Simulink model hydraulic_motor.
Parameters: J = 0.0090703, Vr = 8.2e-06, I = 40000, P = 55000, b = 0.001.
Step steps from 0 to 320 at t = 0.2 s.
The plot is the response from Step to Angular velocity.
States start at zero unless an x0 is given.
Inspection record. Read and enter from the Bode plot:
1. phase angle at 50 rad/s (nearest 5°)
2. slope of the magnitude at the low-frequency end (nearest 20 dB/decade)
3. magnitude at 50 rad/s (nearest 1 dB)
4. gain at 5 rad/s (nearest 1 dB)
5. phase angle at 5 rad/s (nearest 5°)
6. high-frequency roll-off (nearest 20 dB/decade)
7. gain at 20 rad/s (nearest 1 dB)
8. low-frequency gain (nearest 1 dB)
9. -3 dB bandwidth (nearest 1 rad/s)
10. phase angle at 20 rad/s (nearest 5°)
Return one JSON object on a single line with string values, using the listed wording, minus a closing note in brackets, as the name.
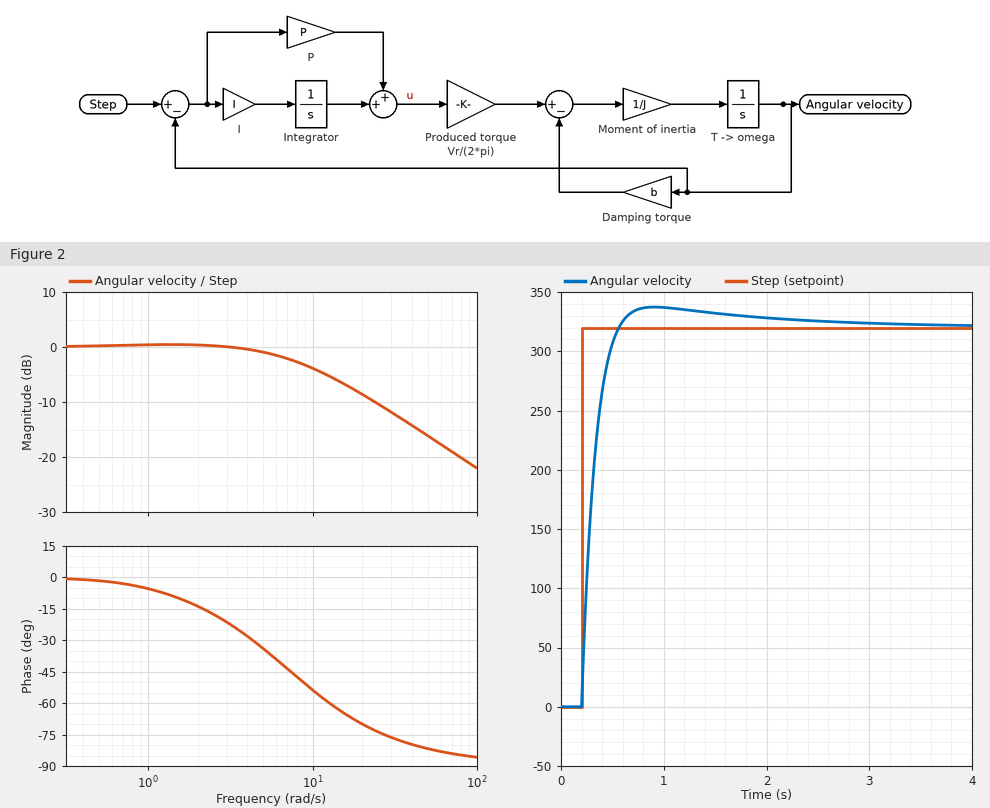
{"phase angle at 50 rad/s": "-80°", "slope of the magnitude at the low-frequency end": "0 dB/decade", "magnitude at 50 rad/s": "-16 dB", "gain at 5 rad/s": "-1 dB", "phase angle at 5 rad/s": "-35°", "high-frequency roll-off": "-20 dB/decade", "gain at 20 rad/s": "-9 dB", "low-frequency gain": "0 dB", "-3 dB bandwidth": "8 rad/s", "phase angle at 20 rad/s": "-70°"}
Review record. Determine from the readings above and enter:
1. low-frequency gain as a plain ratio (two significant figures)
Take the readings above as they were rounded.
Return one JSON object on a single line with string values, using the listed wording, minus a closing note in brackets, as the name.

{"low-frequency gain as a plain ratio": "1.0"}
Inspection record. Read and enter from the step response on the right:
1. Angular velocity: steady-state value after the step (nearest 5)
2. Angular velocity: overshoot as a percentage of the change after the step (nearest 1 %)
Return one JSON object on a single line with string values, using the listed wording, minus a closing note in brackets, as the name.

{"Angular velocity: steady-state value after the step": "320", "Angular velocity: overshoot as a percentage of the change after the step": "5 %"}
